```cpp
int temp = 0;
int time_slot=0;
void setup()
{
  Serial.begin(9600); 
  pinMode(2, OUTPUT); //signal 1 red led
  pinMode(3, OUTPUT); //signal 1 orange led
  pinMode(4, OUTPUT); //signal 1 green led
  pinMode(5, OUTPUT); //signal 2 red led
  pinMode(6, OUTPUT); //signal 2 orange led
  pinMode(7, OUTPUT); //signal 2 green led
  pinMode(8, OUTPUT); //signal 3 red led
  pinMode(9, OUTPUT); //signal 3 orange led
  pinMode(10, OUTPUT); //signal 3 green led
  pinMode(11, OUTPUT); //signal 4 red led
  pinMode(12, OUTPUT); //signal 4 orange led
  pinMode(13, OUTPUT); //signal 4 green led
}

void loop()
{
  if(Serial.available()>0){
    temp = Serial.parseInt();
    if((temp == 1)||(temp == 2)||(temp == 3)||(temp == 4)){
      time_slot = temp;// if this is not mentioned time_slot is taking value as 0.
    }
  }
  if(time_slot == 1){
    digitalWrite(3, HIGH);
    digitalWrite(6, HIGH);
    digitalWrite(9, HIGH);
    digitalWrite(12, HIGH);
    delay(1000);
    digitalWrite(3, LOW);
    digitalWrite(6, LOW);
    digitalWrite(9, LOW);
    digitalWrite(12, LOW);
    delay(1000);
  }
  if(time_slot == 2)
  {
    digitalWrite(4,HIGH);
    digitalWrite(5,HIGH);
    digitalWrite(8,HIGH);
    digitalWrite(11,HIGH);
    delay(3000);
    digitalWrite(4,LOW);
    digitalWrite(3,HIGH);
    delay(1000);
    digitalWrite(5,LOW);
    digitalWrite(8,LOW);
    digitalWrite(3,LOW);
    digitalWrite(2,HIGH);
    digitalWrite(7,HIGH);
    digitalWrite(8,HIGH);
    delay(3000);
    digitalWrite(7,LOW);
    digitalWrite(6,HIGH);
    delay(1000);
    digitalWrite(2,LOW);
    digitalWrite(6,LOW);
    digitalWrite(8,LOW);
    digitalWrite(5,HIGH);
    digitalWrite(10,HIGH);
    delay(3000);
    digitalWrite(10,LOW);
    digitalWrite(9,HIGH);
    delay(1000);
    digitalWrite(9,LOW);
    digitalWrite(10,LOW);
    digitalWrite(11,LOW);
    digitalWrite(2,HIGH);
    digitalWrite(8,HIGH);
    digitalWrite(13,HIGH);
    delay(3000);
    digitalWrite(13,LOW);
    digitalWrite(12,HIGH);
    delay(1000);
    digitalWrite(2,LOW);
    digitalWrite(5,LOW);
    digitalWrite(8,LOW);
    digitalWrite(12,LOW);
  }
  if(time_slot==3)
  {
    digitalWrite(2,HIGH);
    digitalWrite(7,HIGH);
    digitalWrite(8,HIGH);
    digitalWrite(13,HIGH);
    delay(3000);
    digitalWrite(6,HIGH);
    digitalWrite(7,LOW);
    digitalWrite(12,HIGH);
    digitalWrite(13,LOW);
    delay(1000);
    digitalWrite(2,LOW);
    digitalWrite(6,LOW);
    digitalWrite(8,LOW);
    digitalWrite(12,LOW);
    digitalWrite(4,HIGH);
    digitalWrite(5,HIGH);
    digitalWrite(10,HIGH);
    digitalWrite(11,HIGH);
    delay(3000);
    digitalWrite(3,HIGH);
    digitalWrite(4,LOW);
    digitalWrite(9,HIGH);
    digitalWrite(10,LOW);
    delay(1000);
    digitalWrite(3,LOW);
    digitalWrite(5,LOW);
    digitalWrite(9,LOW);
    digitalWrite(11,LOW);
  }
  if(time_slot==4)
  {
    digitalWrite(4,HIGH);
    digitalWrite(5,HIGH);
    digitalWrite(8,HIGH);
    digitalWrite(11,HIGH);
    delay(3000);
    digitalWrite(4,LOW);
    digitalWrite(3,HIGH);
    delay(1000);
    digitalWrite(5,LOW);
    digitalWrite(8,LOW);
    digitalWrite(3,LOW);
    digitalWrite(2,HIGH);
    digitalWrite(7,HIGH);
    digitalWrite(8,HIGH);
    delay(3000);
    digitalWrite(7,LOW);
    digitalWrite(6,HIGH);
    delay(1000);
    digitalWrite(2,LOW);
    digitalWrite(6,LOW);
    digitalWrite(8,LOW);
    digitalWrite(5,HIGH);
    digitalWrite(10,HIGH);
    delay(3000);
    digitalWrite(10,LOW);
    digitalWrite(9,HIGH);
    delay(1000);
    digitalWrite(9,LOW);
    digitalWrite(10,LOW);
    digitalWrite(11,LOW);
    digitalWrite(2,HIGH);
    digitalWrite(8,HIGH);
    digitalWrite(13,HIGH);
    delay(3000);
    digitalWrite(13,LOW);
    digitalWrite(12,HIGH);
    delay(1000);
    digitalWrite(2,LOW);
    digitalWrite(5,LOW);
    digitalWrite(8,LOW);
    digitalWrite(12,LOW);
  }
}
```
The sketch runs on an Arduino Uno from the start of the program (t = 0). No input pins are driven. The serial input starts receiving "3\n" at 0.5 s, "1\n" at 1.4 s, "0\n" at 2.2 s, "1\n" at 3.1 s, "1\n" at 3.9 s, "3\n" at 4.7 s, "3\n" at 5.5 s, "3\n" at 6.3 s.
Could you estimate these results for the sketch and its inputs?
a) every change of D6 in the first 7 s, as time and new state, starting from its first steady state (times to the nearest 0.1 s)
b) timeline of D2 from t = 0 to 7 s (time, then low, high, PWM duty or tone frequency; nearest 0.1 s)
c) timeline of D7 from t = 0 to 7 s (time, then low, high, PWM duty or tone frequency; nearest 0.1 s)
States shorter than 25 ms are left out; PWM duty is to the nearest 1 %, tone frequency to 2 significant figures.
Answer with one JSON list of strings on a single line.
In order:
["0 s low; 3.5 s high; 4.5 s low", "0 s low; 0.5 s high; 4.5 s low", "0 s low; 0.5 s high; 3.5 s low"]
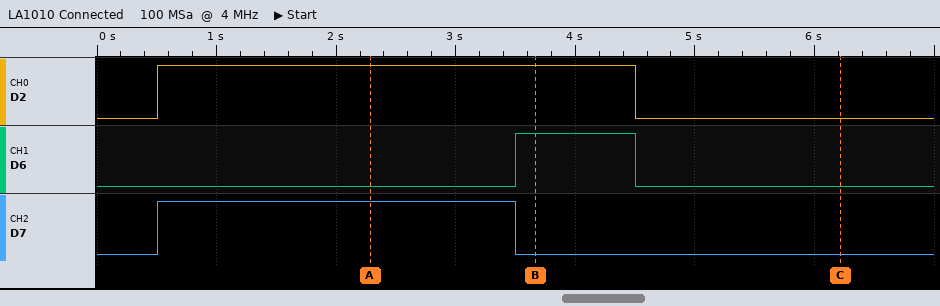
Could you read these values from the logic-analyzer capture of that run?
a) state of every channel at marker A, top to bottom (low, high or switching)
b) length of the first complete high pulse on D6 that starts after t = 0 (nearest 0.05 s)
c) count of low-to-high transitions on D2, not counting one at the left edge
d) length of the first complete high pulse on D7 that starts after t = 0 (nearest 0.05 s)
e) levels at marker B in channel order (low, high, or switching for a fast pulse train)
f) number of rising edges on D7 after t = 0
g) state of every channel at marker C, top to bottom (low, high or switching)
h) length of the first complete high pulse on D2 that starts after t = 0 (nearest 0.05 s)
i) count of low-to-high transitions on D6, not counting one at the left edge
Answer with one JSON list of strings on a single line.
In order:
["D2 high, D6 low, D7 high", "1.00 s", "1", "3.00 s", "D2 high, D6 high, D7 low", "1", "D2 low, D6 low, D7 low", "4.00 s", "1"]
